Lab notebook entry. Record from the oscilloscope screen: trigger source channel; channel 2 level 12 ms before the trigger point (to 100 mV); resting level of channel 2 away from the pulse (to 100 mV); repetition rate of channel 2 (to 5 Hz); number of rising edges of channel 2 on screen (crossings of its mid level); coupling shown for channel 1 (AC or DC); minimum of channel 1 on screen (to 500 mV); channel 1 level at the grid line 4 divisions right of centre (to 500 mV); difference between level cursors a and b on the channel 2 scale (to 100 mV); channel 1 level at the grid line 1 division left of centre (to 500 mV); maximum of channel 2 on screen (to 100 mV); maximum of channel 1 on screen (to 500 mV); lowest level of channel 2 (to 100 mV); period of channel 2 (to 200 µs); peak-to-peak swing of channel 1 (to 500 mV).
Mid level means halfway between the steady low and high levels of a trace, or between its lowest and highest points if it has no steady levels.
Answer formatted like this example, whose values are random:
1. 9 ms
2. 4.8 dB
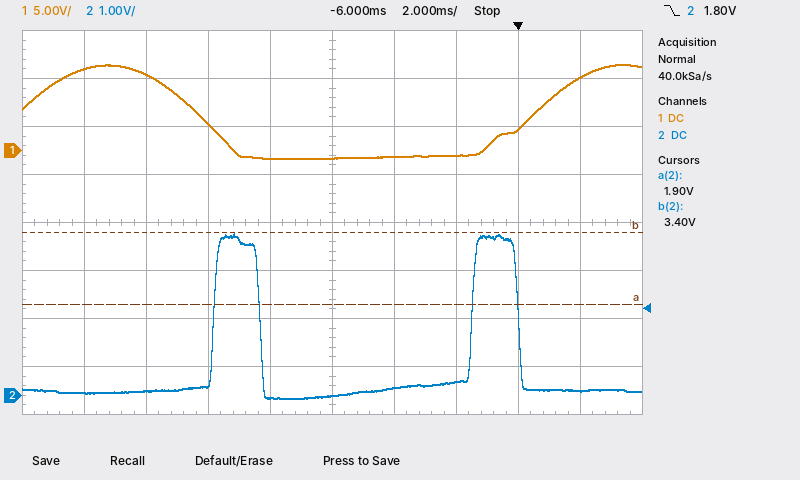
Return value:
1. channel 2
2. 100 mV
3. 100 mV
4. 120 Hz
5. 2
6. DC
7. -1.0 V
8. 7.5 V
9. 1.5 V
10. -1.0 V
11. 3.4 V
12. 9.0 V
13. -100 mV
14. 8.4 ms
15. 10.0 V
